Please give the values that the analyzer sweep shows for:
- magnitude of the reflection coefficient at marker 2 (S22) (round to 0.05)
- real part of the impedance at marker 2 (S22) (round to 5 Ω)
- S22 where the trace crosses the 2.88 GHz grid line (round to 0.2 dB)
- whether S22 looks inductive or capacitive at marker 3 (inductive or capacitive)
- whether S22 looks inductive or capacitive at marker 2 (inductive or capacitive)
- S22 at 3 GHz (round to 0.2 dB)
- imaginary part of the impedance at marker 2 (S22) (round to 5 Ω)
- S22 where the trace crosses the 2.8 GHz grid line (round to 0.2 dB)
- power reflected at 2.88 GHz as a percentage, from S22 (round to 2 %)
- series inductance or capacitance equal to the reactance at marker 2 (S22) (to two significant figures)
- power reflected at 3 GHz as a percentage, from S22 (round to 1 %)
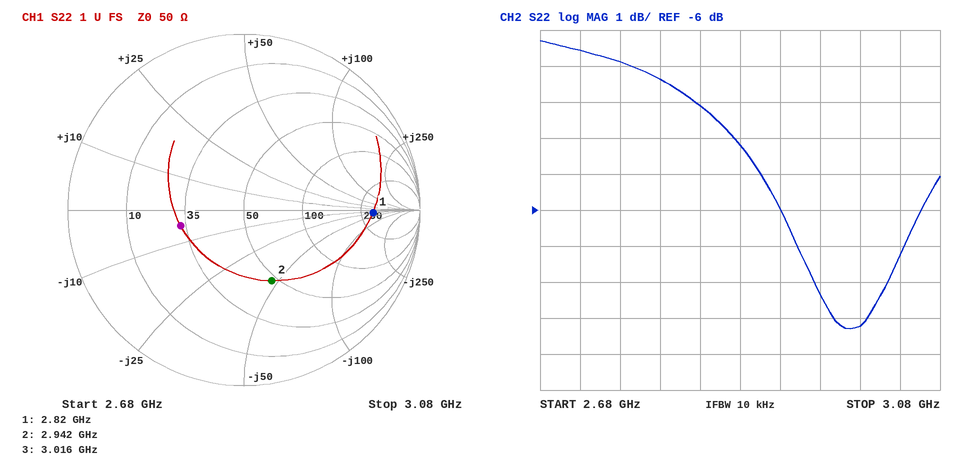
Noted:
0.45
45 Ω
-4.2 dB
capacitive
capacitive
-9.2 dB
-45 Ω
-2.4 dB
38 %
1.2 pF
12 %
